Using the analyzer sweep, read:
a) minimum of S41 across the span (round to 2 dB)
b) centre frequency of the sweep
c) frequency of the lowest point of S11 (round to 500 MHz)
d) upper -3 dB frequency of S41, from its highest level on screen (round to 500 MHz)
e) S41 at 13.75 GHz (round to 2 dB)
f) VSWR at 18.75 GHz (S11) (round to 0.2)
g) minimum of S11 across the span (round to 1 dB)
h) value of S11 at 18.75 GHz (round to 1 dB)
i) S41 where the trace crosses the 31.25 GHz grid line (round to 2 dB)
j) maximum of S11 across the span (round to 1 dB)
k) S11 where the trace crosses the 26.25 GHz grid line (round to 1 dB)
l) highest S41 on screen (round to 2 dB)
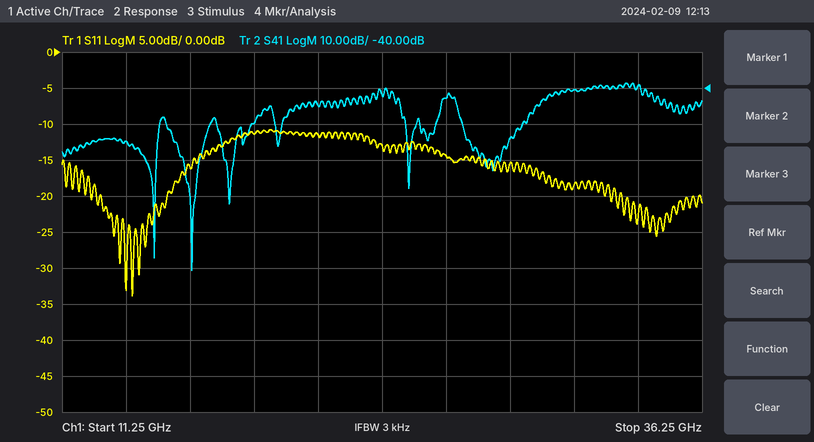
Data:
-90 dB
23.75 GHz
14.0 GHz
34.0 GHz
-54 dB
1.8
-34 dB
-11 dB
-40 dB
-11 dB
-14 dB
-38 dB
